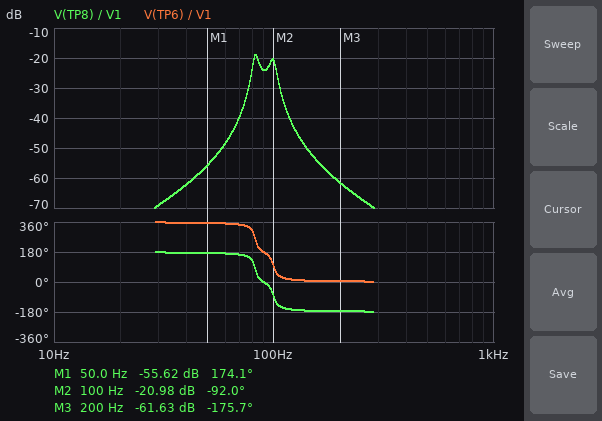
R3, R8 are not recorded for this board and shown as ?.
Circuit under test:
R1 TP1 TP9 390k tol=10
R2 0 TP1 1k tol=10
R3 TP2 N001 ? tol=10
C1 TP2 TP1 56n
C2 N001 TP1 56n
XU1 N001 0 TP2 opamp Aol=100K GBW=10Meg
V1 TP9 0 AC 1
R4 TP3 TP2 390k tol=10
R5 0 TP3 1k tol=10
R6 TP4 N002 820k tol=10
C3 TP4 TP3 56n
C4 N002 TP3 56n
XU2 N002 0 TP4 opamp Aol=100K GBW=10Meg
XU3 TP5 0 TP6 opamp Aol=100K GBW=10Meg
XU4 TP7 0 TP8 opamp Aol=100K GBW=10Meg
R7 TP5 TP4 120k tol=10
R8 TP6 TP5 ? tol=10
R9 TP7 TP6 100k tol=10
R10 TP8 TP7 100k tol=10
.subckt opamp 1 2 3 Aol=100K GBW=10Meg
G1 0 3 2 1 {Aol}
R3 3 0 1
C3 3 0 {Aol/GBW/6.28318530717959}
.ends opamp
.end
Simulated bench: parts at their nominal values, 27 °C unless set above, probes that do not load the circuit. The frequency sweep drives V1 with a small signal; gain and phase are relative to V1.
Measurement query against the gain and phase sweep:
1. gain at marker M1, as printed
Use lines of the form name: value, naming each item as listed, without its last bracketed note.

gain at marker M1, as printed: -55.62 dB
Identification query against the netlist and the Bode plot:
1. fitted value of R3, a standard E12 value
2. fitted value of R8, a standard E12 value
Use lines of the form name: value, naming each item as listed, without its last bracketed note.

fitted value of R3, a standard E12 value: 1.2 MΩ
fitted value of R8, a standard E12 value: 47 kΩ
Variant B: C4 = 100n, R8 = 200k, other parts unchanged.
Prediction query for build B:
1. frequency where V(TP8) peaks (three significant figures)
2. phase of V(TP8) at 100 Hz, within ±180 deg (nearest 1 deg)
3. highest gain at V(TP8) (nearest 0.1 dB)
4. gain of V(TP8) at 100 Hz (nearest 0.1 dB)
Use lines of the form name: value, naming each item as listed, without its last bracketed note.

frequency where V(TP8) peaks: 81.4 Hz
phase of V(TP8) at 100 Hz, within ±180 deg: -165 deg
highest gain at V(TP8): 1.7 dB
gain of V(TP8) at 100 Hz: -24.5 dB
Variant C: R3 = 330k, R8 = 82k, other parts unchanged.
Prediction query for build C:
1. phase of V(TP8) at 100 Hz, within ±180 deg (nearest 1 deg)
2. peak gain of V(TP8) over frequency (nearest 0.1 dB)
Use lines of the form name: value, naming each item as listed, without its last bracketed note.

phase of V(TP8) at 100 Hz, within ±180 deg: 73 deg
peak gain of V(TP8) over frequency: -29.1 dB
